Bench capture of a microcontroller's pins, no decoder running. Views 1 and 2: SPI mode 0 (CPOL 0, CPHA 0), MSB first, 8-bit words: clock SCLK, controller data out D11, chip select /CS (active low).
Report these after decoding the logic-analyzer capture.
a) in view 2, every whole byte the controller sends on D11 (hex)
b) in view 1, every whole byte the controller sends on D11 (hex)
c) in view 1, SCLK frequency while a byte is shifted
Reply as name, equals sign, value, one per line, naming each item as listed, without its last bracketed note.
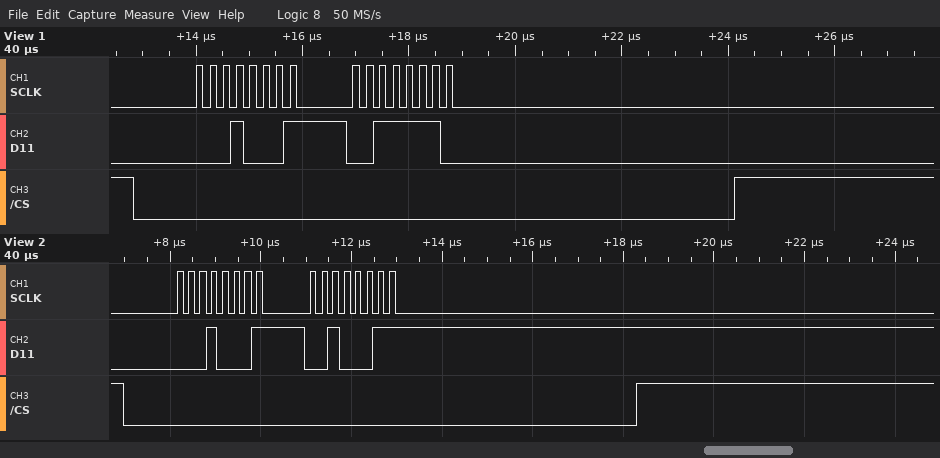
in view 2, every whole byte the controller sends on D11 = 11 23
in view 1, every whole byte the controller sends on D11 = 11 3E
in view 1, SCLK frequency while a byte is shifted = 4 MHz
